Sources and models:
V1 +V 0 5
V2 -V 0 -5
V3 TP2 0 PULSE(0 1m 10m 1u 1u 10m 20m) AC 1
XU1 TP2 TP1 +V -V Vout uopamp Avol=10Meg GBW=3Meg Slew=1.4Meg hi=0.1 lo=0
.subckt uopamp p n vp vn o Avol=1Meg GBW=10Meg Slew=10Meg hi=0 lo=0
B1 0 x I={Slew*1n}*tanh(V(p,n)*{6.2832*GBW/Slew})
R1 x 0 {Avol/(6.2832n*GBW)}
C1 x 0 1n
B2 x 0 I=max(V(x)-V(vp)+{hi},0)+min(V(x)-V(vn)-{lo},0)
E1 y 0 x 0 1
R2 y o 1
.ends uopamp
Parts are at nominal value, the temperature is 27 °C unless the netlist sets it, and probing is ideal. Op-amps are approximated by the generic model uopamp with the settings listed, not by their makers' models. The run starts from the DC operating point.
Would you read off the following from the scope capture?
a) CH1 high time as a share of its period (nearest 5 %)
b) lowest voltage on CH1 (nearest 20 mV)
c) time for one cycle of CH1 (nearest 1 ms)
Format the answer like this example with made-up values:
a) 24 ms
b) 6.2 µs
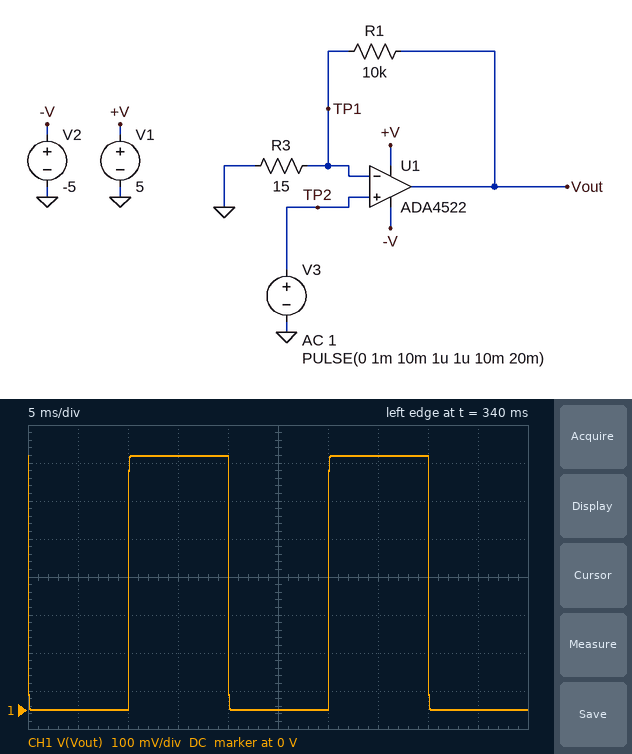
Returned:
a) 50 %
b) 0 V
c) 20 ms
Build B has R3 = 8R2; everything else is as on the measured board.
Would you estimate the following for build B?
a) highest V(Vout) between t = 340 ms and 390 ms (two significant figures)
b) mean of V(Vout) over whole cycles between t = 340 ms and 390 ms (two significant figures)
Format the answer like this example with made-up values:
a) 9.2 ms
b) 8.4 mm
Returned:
a) 1.2 V
b) 610 mV
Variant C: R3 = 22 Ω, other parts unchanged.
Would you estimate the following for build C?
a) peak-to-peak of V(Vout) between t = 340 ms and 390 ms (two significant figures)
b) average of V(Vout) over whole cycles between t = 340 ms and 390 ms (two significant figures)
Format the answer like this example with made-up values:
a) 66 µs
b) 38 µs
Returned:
a) 460 mV
b) 230 mV
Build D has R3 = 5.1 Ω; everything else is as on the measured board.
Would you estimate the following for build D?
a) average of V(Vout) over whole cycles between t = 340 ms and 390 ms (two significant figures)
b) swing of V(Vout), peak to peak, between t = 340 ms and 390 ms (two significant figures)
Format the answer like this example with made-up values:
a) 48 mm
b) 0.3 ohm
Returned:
a) 980 mV
b) 2.0 V
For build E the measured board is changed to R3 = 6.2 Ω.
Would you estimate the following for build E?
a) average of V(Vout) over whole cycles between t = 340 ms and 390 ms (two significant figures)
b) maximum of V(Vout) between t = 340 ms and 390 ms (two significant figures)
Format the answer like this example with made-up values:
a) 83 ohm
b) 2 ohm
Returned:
a) 810 mV
b) 1.6 V
